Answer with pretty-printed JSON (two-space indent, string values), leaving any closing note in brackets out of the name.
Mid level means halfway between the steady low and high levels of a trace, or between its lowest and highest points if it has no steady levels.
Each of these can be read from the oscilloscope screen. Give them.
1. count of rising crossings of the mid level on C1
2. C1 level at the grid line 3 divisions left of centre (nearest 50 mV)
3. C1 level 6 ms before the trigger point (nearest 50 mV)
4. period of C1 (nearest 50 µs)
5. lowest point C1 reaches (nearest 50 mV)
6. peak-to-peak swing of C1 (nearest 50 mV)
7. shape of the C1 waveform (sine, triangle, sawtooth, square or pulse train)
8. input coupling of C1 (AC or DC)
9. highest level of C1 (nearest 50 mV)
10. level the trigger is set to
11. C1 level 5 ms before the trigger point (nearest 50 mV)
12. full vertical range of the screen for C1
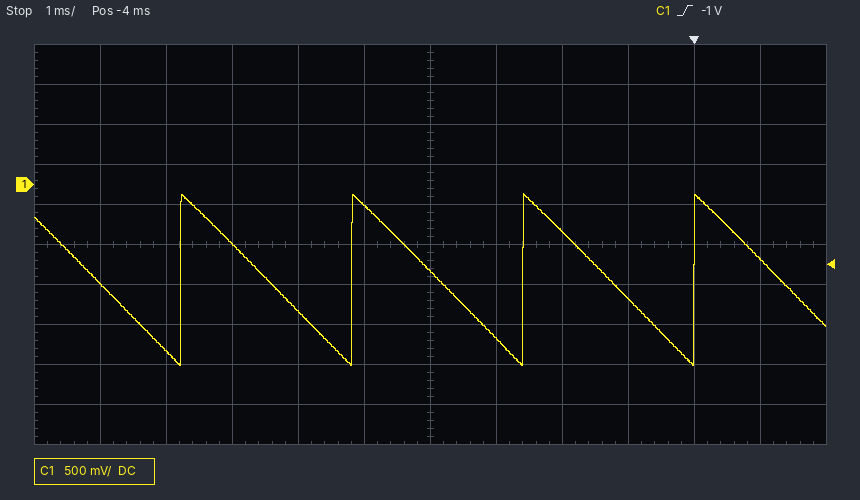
{
  "count of rising crossings of the mid level on C1": "4",
  "C1 level at the grid line 3 divisions left of centre": "-750 mV",
  "C1 level 6 ms before the trigger point": "-1.60 V",
  "period of C1": "2.60 ms",
  "lowest point C1 reaches": "-2.25 V",
  "peak-to-peak swing of C1": "2.15 V",
  "shape of the C1 waveform": "sawtooth",
  "input coupling of C1": "DC",
  "highest level of C1": "-100 mV",
  "level the trigger is set to": "-1 V",
  "C1 level 5 ms before the trigger point": "-250 mV",
  "full vertical range of the screen for C1": "5 V"
}
